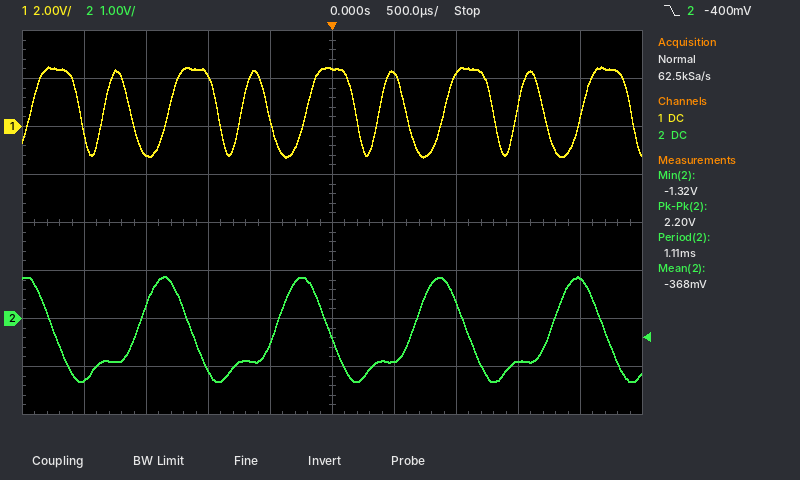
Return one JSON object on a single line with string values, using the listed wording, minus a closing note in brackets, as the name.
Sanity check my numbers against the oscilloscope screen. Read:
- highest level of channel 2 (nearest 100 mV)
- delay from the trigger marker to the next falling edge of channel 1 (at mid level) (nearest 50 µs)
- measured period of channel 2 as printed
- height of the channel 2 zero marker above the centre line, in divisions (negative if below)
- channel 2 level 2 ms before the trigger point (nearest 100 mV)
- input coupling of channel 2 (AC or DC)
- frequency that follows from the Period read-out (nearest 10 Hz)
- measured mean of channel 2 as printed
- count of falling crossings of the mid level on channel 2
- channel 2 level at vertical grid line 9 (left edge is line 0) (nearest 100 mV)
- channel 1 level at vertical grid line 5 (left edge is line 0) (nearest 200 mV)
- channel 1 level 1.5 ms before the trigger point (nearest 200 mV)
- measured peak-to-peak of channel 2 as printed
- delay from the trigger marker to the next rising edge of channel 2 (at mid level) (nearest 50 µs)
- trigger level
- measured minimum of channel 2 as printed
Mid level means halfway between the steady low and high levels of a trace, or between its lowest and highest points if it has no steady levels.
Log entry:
{"highest level of channel 2": "900 mV", "delay from the trigger marker to the next falling edge of channel 1 (at mid level)": "200 µs", "measured period of channel 2 as printed": "1.11 ms", "height of the channel 2 zero marker above the centre line, in divisions": "-2.0 div", "channel 2 level 2 ms before the trigger point": "-1.3 V", "input coupling of channel 2": "DC", "frequency that follows from the Period read-out": "900 Hz", "measured mean of channel 2 as printed": "-368 mV", "count of falling crossings of the mid level on channel 2": "5", "channel 2 level at vertical grid line 9 (left edge is line 0)": "800 mV", "channel 1 level at vertical grid line 5 (left edge is line 0)": "2.4 V", "channel 1 level 1.5 ms before the trigger point": "-1.2 V", "measured peak-to-peak of channel 2 as printed": "2.20 V", "delay from the trigger marker to the next rising edge of channel 2 (at mid level)": "650 µs", "trigger level": "-400 mV", "measured minimum of channel 2 as printed": "-1.32 V"}
